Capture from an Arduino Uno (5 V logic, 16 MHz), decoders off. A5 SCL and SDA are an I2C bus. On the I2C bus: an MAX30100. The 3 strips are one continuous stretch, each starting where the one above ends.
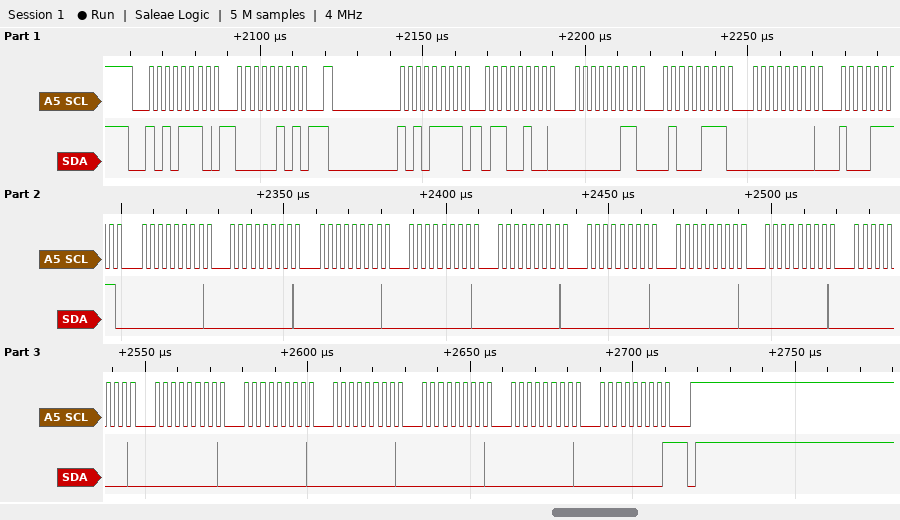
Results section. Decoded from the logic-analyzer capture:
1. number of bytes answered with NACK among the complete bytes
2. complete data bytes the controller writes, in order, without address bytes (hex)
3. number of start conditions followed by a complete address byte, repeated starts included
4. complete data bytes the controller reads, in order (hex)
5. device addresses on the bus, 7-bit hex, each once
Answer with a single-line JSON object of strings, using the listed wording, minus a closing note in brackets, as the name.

{"number of bytes answered with NACK among the complete bytes": "1", "complete data bytes the controller writes, in order, without address bytes": "05", "number of start conditions followed by a complete address byte, repeated starts included": "2", "complete data bytes the controller reads, in order": "64 03 47 00 8F 00 00 00 00 00 00 00 00 00 00 00 00 00 00 00", "device addresses on the bus, 7-bit hex, each once": "0x57"}
